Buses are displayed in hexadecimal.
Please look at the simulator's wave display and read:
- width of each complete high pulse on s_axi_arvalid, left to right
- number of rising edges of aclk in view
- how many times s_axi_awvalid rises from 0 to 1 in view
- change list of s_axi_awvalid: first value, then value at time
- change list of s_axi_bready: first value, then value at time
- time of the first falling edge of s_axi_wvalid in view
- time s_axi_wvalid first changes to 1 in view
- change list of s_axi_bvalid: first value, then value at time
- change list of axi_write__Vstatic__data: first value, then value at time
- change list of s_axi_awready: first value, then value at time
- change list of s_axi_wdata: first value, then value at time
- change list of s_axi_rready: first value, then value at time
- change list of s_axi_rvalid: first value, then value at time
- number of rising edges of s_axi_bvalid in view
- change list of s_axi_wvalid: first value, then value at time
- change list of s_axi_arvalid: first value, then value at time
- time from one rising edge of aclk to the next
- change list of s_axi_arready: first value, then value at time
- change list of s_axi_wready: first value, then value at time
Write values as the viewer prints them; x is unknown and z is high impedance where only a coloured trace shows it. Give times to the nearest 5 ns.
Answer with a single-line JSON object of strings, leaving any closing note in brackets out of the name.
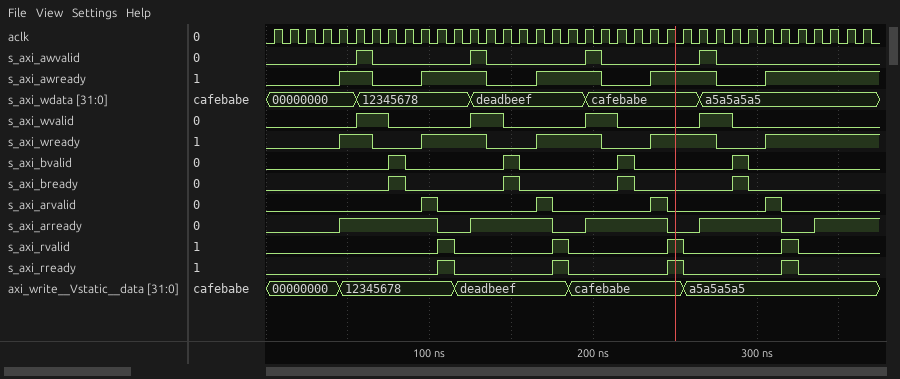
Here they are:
{"width of each complete high pulse on s_axi_arvalid, left to right": "10 ns, 10 ns, 10 ns, 10 ns", "number of rising edges of aclk in view": "37", "how many times s_axi_awvalid rises from 0 to 1 in view": "4", "change list of s_axi_awvalid: first value, then value at time": "0, 1 at 55 ns, 0 at 65 ns, 1 at 125 ns, 0 at 135 ns, 1 at 195 ns, 0 at 205 ns, 1 at 265 ns, 0 at 275 ns", "change list of s_axi_bready: first value, then value at time": "0, 1 at 75 ns, 0 at 85 ns, 1 at 145 ns, 0 at 155 ns, 1 at 215 ns, 0 at 225 ns, 1 at 285 ns, 0 at 295 ns", "time of the first falling edge of s_axi_wvalid in view": "75 ns", "time s_axi_wvalid first changes to 1 in view": "55 ns", "change list of s_axi_bvalid: first value, then value at time": "0, 1 at 75 ns, 0 at 85 ns, 1 at 145 ns, 0 at 155 ns, 1 at 215 ns, 0 at 225 ns, 1 at 285 ns, 0 at 295 ns", "change list of axi_write__Vstatic__data: first value, then value at time": "00000000, 12345678 at 45 ns, deadbeef at 115 ns, cafebabe at 185 ns, a5a5a5a5 at 255 ns", "change list of s_axi_awready: first value, then value at time": "0, 1 at 45 ns, 0 at 65 ns, 1 at 95 ns, 0 at 135 ns, 1 at 165 ns, 0 at 205 ns, 1 at 235 ns, 0 at 275 ns, 1 at 305 ns", "change list of s_axi_wdata: first value, then value at time": "00000000, 12345678 at 55 ns, deadbeef at 125 ns, cafebabe at 195 ns, a5a5a5a5 at 265 ns", "change list of s_axi_rready: first value, then value at time": "0, 1 at 105 ns, 0 at 115 ns, 1 at 175 ns, 0 at 185 ns, 1 at 245 ns, 0 at 255 ns, 1 at 315 ns, 0 at 325 ns", "change list of s_axi_rvalid: first value, then value at time": "0, 1 at 105 ns, 0 at 115 ns, 1 at 175 ns, 0 at 185 ns, 1 at 245 ns, 0 at 255 ns, 1 at 315 ns, 0 at 325 ns", "number of rising edges of s_axi_bvalid in view": "4", "change list of s_axi_wvalid: first value, then value at time": "0, 1 at 55 ns, 0 at 75 ns, 1 at 125 ns, 0 at 145 ns, 1 at 195 ns, 0 at 215 ns, 1 at 265 ns, 0 at 285 ns", "change list of s_axi_arvalid: first value, then value at time": "0, 1 at 95 ns, 0 at 105 ns, 1 at 165 ns, 0 at 175 ns, 1 at 235 ns, 0 at 245 ns, 1 at 305 ns, 0 at 315 ns", "time from one rising edge of aclk to the next": "10 ns", "change list of s_axi_arready: first value, then value at time": "0, 1 at 45 ns, 0 at 105 ns, 1 at 125 ns, 0 at 175 ns, 1 at 195 ns, 0 at 245 ns, 1 at 265 ns, 0 at 315 ns, 1 at 335 ns", "change list of s_axi_wready: first value, then value at time": "0, 1 at 45 ns, 0 at 65 ns, 1 at 95 ns, 0 at 135 ns, 1 at 165 ns, 0 at 205 ns, 1 at 235 ns, 0 at 275 ns, 1 at 305 ns"}
